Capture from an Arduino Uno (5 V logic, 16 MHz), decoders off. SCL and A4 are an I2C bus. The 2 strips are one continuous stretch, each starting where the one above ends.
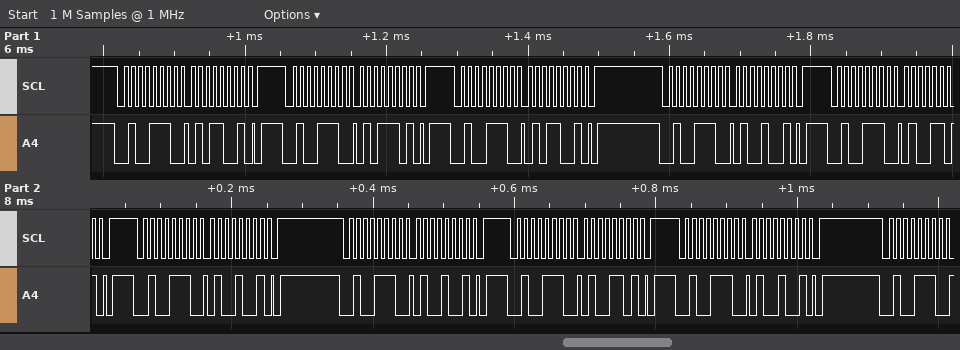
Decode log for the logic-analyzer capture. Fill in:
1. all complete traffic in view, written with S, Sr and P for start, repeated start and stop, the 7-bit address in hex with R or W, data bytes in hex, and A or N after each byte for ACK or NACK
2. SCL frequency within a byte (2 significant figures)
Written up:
S 27W A 59 A P S 27W A 5D A P S 27W A 59 A P S 27W A 49 A P S 27W A 4D A P S 27W A 49 A P S 27W A 49 A P S 27W A 4D A P S 27W A 49 A P S 27W A
100 kHz
